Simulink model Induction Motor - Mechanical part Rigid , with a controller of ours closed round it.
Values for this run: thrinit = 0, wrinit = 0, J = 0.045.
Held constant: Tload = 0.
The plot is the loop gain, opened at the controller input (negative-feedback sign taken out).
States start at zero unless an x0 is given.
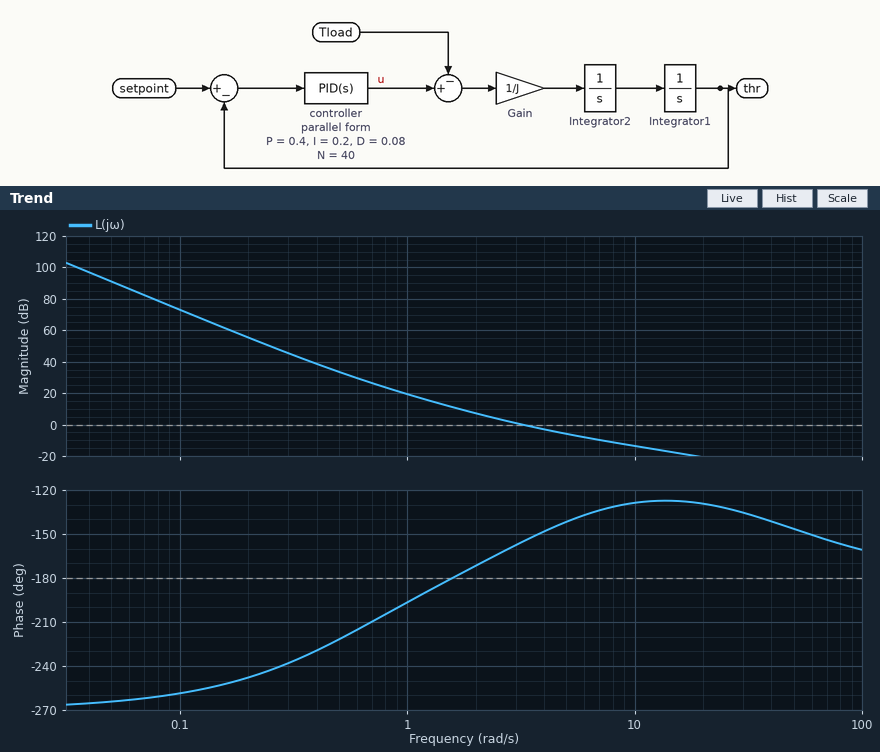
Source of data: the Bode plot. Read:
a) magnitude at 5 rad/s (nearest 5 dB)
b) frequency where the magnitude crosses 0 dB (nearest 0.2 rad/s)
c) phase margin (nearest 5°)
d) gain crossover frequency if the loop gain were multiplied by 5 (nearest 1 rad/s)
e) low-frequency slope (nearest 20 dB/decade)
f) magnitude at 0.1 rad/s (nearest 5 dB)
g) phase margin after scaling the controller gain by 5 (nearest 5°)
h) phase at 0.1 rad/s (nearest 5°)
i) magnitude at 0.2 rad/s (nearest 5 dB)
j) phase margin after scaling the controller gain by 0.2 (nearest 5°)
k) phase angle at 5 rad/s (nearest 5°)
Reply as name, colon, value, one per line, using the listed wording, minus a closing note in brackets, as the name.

magnitude at 5 rad/s: -5 dB
frequency where the magnitude crosses 0 dB: 3.2 rad/s
phase margin: 25°
gain crossover frequency if the loop gain were multiplied by 5: 10 rad/s
low-frequency slope: -60 dB/decade
magnitude at 0.1 rad/s: 75 dB
phase margin after scaling the controller gain by 5: 50°
phase at 0.1 rad/s: -260°
magnitude at 0.2 rad/s: 55 dB
phase margin after scaling the controller gain by 0.2: -5°
phase angle at 5 rad/s: -140°
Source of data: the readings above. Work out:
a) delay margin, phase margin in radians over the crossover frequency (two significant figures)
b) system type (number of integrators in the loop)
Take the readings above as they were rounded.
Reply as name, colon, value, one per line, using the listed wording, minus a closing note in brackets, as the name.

delay margin, phase margin in radians over the crossover frequency: 0.14 s
system type: 3
